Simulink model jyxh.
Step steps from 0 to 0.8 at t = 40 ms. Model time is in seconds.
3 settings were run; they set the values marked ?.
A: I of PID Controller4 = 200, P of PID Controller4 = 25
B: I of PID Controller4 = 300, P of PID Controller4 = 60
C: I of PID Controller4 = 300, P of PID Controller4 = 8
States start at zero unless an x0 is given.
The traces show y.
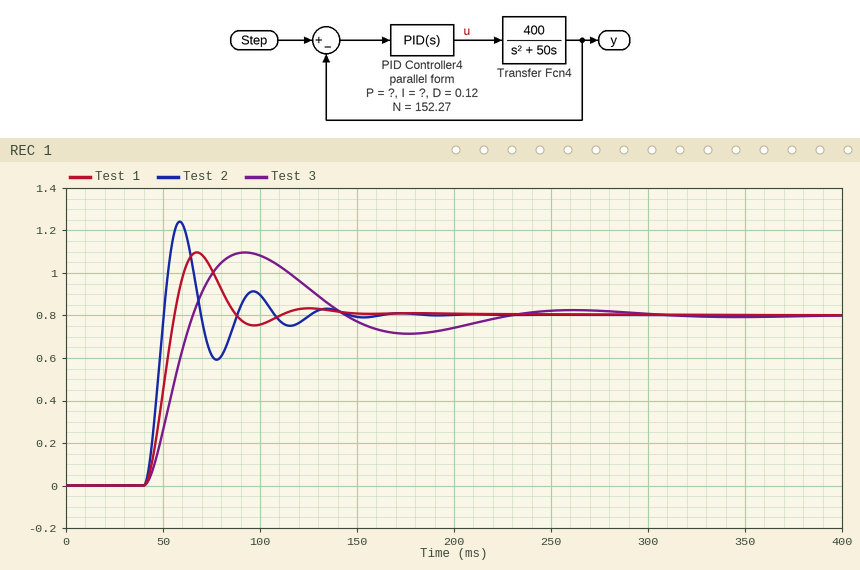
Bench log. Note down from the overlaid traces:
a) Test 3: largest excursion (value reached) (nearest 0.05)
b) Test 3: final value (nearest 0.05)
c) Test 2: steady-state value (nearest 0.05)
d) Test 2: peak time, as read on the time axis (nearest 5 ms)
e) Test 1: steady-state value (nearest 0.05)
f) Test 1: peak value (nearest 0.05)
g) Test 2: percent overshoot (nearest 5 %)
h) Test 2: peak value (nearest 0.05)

1.10
0.80
0.80
60 ms
0.80
1.10
55 %
1.25
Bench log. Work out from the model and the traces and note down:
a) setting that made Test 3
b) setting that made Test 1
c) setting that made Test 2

C
A
B
